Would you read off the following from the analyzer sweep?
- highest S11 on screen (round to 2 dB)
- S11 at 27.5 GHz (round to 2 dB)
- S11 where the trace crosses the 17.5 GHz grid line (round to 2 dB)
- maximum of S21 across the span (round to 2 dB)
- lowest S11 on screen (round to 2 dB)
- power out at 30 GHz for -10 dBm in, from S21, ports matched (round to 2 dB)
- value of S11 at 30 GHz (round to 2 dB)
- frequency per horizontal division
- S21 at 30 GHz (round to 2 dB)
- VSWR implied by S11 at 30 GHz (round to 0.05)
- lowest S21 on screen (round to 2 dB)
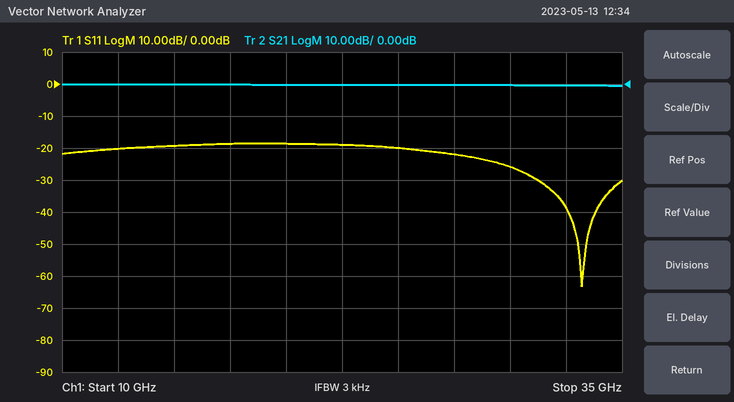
-18 dB
-22 dB
-18 dB
0 dB
-64 dB
-10 dBm
-26 dB
2.5 GHz
0 dB
1.10
0 dB
